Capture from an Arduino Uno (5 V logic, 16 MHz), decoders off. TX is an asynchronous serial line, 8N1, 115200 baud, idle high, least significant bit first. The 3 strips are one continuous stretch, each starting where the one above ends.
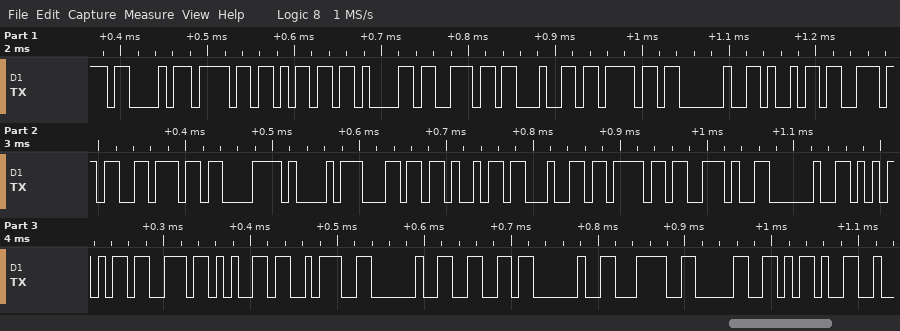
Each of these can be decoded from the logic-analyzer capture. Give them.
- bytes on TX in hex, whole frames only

0x43 0x6F 0x6D 0x61 0x6E 0x64 0x6F 0x20 0x69 0x6E 0x76 0xC3 0xA1 0x6C 0x69 0x64 0x6F 0x2E 0x20 0x55 0x73 0x65 0x3A 0x20 0x66 0x20 0x3C 0x30 0x2D
